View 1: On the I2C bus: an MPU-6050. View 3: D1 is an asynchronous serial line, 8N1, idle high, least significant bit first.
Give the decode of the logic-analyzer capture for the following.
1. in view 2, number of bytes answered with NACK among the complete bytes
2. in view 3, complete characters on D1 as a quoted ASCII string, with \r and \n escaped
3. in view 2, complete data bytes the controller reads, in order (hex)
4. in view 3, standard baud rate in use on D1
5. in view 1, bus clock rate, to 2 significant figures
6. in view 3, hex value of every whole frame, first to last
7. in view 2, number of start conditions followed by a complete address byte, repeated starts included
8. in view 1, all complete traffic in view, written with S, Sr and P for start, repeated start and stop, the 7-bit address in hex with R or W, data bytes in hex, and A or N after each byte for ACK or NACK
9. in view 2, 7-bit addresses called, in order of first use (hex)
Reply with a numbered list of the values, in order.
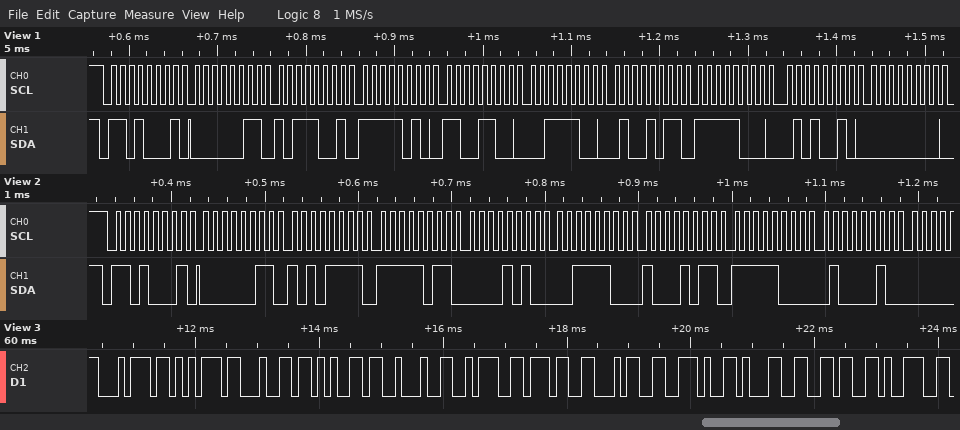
1. 0
2. "tude\":74.169"
3. 03 AF FB 0A 3C 8B F8 42
4. 9600 baud
5. 100 kHz
6. 74 75 64 65 22 3A 37 34 2E 31 36 39
7. 1
8. S 68R A 03 A B9 A FA A CC A 3C A 4B A F8 A 52 A 00 A
9. 0x68
